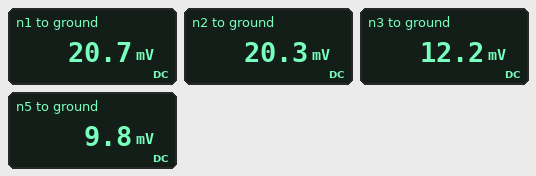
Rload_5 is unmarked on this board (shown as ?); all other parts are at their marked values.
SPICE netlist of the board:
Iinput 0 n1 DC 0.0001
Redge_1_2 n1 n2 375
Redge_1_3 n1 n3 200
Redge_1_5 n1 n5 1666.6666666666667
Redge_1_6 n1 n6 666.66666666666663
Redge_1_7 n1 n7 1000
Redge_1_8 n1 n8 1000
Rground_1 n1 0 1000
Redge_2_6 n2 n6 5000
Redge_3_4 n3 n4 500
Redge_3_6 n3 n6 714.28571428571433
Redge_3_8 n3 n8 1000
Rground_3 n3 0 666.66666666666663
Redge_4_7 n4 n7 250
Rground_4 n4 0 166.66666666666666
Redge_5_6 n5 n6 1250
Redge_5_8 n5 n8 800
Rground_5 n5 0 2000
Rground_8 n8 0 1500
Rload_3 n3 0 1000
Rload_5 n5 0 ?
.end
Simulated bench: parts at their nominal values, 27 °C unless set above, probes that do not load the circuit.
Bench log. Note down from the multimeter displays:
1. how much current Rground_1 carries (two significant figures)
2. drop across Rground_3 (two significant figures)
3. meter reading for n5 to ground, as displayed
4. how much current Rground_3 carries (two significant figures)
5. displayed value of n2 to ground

21 µA
12 mV
9.8 mV
18 µA
20.3 mV
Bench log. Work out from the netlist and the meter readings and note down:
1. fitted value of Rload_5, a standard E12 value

1.2 kΩ
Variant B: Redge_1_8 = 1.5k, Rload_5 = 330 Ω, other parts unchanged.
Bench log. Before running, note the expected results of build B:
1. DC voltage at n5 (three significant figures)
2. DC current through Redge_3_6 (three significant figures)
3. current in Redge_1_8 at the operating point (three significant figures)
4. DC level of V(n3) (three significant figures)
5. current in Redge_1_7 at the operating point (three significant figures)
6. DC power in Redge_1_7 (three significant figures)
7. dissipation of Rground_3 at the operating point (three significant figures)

5.49 mV
3.38 µA
7.34 µA
11.4 mV
12.3 µA
152 nW
196 nW
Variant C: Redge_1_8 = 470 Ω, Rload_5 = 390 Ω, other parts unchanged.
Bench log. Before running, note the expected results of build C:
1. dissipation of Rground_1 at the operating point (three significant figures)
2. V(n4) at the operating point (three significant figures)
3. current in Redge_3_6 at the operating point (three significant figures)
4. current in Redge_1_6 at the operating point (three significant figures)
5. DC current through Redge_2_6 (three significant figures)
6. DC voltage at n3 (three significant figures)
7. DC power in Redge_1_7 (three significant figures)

355 nW
4.26 mV
3.26 µA
7.94 µA
985 nA
11.2 mV
136 nW
